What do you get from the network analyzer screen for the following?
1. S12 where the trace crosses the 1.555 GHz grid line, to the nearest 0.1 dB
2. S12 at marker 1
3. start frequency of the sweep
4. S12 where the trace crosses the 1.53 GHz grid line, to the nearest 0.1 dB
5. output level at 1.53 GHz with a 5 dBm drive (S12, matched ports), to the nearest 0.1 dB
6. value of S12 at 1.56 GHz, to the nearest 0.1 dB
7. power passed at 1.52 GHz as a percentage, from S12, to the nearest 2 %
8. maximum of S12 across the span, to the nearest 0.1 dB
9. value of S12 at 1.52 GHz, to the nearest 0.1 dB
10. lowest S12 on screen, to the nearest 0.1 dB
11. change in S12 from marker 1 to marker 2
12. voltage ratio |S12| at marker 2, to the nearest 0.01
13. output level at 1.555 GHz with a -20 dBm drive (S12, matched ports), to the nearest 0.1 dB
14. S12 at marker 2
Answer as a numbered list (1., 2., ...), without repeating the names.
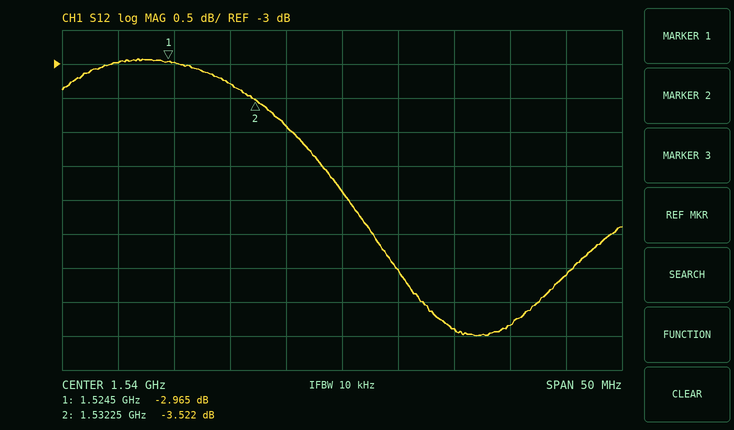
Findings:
1. -6.8 dB
2. -2.965 dB
3. 1.515 GHz
4. -3.3 dB
5. 1.7 dBm
6. -6.1 dB
7. 50 %
8. -2.9 dB
9. -3.0 dB
10. -7.0 dB
11. -0.557 dB
12. 0.67
13. -26.8 dBm
14. -3.522 dB
